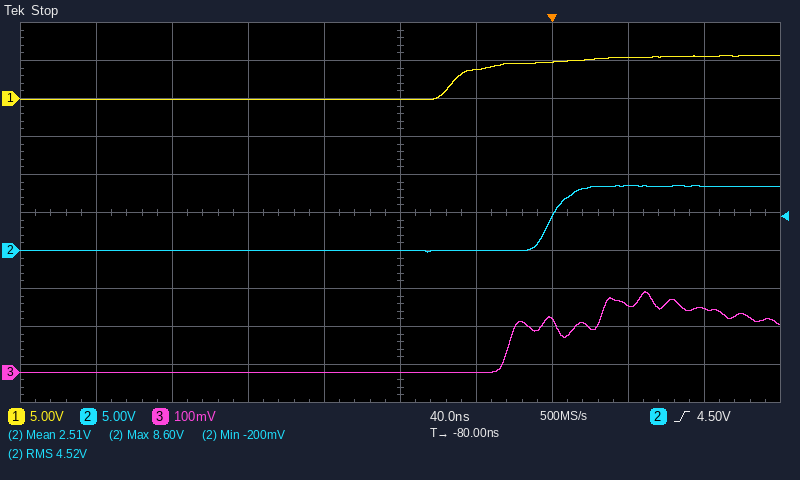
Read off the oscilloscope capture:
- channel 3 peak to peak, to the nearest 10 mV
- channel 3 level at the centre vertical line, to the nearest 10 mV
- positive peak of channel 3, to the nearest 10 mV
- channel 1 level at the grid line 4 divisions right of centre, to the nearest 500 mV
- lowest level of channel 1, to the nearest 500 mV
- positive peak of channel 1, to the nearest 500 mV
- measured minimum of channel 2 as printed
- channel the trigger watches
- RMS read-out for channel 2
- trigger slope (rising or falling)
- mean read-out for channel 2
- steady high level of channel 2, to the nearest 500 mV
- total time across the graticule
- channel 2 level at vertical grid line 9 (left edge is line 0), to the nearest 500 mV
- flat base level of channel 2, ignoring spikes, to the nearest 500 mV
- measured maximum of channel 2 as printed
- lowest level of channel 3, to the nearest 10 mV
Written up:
210 mV
0 mV
210 mV
5.5 V
0.0 V
5.5 V
-200 mV
channel 2
4.52 V
rising
2.51 V
8.5 V
400 ns
8.5 V
0.0 V
8.60 V
0 mV
